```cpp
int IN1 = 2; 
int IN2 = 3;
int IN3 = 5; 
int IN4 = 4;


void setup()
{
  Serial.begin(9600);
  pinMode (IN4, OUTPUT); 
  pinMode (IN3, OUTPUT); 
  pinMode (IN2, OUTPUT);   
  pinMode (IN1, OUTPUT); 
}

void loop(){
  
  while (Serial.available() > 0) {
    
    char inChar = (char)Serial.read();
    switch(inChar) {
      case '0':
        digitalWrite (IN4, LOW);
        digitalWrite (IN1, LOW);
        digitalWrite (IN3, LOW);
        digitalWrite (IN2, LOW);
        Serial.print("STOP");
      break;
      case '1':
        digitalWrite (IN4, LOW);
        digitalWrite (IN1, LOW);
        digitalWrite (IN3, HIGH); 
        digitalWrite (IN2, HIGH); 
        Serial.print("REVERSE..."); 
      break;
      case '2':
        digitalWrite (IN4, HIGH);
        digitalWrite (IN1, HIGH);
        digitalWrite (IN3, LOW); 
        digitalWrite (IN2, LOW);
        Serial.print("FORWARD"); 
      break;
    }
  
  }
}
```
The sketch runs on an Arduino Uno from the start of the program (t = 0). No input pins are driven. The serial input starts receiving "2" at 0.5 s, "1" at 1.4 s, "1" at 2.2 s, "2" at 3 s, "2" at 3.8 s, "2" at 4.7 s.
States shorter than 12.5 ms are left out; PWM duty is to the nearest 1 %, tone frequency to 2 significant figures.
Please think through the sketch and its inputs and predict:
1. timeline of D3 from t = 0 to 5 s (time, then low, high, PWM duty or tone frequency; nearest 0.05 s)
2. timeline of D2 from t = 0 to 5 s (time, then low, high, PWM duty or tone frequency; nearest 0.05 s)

0 s low; 1.4 s high; 3 s low
0 s low; 0.5 s high; 1.4 s low; 3 s high
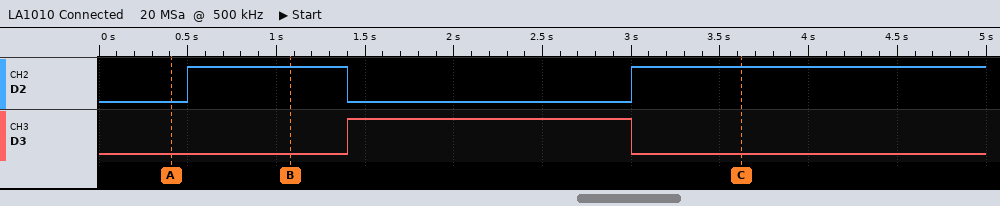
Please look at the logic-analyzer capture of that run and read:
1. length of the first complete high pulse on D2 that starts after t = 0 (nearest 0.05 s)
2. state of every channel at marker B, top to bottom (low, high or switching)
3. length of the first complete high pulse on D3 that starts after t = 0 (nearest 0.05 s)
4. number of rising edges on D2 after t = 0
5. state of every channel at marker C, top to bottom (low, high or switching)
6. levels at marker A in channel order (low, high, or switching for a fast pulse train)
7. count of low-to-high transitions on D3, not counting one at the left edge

0.90 s
D2 high, D3 low
1.60 s
2
D2 high, D3 low
D2 low, D3 low
1
